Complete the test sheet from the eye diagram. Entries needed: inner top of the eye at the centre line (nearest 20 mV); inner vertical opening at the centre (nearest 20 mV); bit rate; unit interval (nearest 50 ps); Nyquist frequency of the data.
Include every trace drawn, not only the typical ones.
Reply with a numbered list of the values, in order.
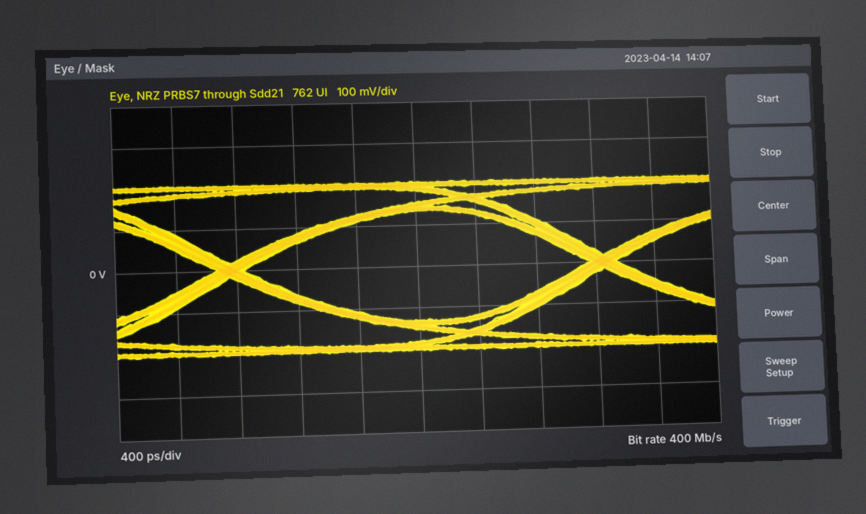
1. 140 mV
2. 260 mV
3. 400 Mb/s
4. 2.50 ns
5. 200 MHz
